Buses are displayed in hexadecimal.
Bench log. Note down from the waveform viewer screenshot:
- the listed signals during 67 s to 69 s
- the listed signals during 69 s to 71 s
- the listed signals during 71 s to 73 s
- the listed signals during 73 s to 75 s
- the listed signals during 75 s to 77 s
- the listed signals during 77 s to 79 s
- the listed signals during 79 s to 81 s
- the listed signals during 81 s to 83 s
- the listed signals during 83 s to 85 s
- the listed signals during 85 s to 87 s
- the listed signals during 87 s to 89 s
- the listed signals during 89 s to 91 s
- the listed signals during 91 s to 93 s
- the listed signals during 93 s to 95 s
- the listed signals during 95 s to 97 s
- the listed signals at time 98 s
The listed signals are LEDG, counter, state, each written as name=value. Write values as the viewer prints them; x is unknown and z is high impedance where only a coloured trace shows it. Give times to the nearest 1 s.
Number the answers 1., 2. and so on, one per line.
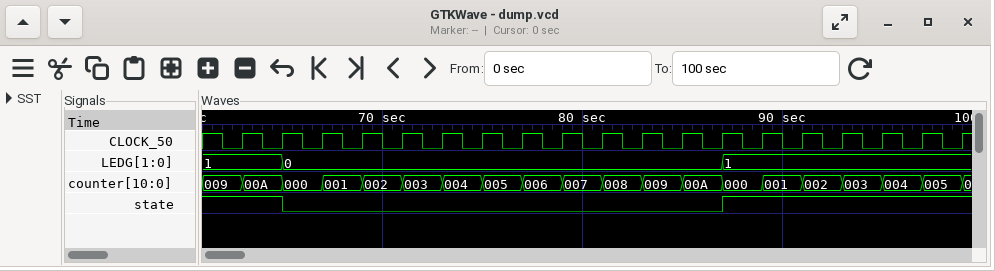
1. LEDG=0, counter=001, state=0
2. LEDG=0, counter=002, state=0
3. LEDG=0, counter=003, state=0
4. LEDG=0, counter=004, state=0
5. LEDG=0, counter=005, state=0
6. LEDG=0, counter=006, state=0
7. LEDG=0, counter=007, state=0
8. LEDG=0, counter=008, state=0
9. LEDG=0, counter=009, state=0
10. LEDG=0, counter=00A, state=0
11. LEDG=1, counter=000, state=1
12. LEDG=1, counter=001, state=1
13. LEDG=1, counter=002, state=1
14. LEDG=1, counter=003, state=1
15. LEDG=1, counter=004, state=1
16. LEDG=1, counter=005, state=1
